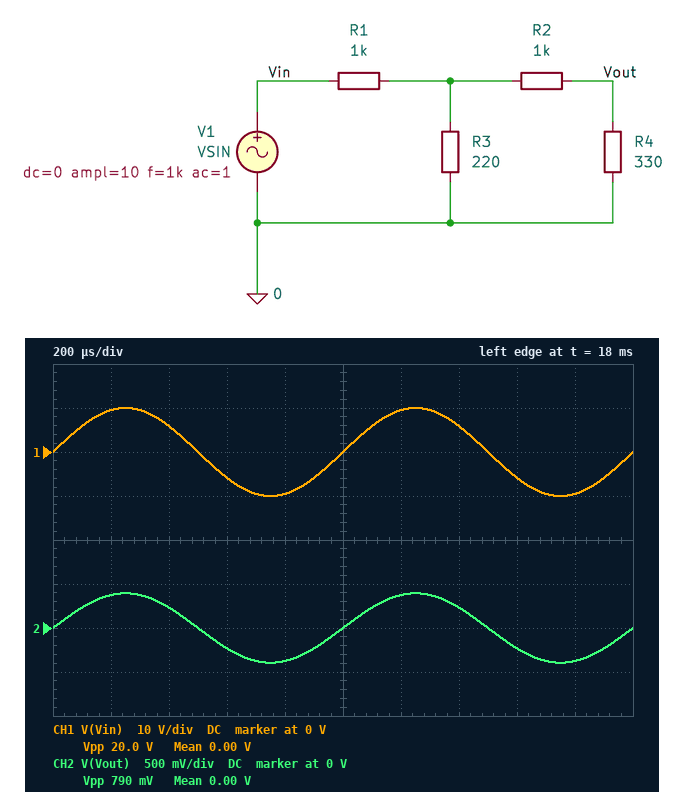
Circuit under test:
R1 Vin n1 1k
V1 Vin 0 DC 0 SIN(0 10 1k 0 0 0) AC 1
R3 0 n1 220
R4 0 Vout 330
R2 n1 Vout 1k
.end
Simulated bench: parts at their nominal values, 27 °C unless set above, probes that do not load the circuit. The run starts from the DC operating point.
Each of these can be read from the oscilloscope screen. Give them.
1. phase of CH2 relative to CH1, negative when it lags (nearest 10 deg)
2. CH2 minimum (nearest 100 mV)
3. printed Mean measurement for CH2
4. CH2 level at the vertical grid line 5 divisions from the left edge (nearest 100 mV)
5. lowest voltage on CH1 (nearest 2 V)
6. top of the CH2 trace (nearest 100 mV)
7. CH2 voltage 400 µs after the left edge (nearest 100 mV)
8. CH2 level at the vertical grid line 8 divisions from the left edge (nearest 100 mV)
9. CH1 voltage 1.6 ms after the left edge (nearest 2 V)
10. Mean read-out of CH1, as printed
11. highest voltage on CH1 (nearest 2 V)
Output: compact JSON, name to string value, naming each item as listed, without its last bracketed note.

{"phase of CH2 relative to CH1, negative when it lags": "0 deg", "CH2 minimum": "-400 mV", "printed Mean measurement for CH2": "0.00 V", "CH2 level at the vertical grid line 5 divisions from the left edge": "0 V", "lowest voltage on CH1": "-10 V", "top of the CH2 trace": "400 mV", "CH2 voltage 400 µs after the left edge": "200 mV", "CH2 level at the vertical grid line 8 divisions from the left edge": "-200 mV", "CH1 voltage 1.6 ms after the left edge": "-6 V", "Mean read-out of CH1, as printed": "0.00 V", "highest voltage on CH1": "10 V"}
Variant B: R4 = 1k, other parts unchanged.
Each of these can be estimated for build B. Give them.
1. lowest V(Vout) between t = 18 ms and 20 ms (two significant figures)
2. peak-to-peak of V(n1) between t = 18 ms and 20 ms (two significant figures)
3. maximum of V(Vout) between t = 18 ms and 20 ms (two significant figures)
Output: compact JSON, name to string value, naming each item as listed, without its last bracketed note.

{"lowest V(Vout) between t = 18 ms and 20 ms": "-830 mV", "peak-to-peak of V(n1) between t = 18 ms and 20 ms": "3.3 V", "maximum of V(Vout) between t = 18 ms and 20 ms": "830 mV"}
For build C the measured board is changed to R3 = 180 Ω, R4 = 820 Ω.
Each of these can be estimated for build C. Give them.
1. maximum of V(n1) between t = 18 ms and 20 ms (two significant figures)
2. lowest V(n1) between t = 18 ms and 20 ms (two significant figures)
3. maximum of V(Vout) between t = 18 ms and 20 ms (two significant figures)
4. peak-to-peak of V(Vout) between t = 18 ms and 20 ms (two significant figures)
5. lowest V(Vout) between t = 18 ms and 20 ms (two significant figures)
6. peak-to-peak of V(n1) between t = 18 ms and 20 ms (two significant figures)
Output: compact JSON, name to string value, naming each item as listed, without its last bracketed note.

{"maximum of V(n1) between t = 18 ms and 20 ms": "1.4 V", "lowest V(n1) between t = 18 ms and 20 ms": "-1.4 V", "maximum of V(Vout) between t = 18 ms and 20 ms": "630 mV", "peak-to-peak of V(Vout) between t = 18 ms and 20 ms": "1.3 V", "lowest V(Vout) between t = 18 ms and 20 ms": "-630 mV", "peak-to-peak of V(n1) between t = 18 ms and 20 ms": "2.8 V"}
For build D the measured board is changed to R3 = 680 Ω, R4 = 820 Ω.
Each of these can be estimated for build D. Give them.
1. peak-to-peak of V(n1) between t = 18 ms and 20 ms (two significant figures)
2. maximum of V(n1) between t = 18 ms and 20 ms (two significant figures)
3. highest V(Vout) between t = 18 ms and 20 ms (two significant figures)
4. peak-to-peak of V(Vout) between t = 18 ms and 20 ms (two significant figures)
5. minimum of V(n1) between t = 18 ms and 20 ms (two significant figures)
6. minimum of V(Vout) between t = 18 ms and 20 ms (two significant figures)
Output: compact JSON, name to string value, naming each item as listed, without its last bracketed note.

{"peak-to-peak of V(n1) between t = 18 ms and 20 ms": "6.6 V", "maximum of V(n1) between t = 18 ms and 20 ms": "3.3 V", "highest V(Vout) between t = 18 ms and 20 ms": "1.5 V", "peak-to-peak of V(Vout) between t = 18 ms and 20 ms": "3.0 V", "minimum of V(n1) between t = 18 ms and 20 ms": "-3.3 V", "minimum of V(Vout) between t = 18 ms and 20 ms": "-1.5 V"}
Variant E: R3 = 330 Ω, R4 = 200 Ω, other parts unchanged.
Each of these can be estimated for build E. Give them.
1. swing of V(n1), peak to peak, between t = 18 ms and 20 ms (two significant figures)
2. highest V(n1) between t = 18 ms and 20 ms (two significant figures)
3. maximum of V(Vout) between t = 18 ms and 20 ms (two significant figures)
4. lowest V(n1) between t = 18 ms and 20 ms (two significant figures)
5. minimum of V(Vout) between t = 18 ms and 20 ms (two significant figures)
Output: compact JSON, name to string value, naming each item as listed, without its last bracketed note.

{"swing of V(n1), peak to peak, between t = 18 ms and 20 ms": "4.1 V", "highest V(n1) between t = 18 ms and 20 ms": "2.1 V", "maximum of V(Vout) between t = 18 ms and 20 ms": "340 mV", "lowest V(n1) between t = 18 ms and 20 ms": "-2.1 V", "minimum of V(Vout) between t = 18 ms and 20 ms": "-340 mV"}
